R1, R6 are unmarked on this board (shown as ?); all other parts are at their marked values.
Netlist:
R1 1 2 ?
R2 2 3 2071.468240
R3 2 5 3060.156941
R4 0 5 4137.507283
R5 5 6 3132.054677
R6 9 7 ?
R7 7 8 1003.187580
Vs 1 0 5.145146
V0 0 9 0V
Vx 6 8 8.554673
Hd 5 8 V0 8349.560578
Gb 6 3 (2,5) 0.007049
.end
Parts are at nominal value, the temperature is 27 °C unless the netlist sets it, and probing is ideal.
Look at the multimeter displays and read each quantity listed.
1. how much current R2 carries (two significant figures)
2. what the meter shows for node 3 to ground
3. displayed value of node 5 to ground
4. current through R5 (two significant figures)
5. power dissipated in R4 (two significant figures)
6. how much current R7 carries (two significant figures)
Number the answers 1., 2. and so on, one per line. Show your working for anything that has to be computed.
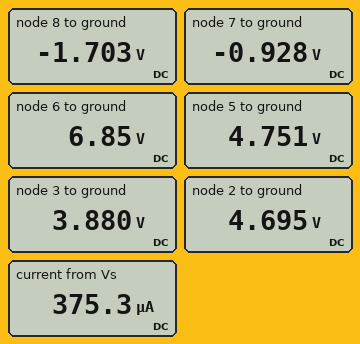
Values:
1. (4.695 V - 3.88 V) / 2.071 kΩ = 390 µA
2. 3.880 V
3. 4.751 V
4. (6.85 V - 4.751 V) / 3.132 kΩ = 670 µA
5. (4.751 V)^2 / 4.138 kΩ = 5.5 mW
6. (-928 mV - (-1.703 V)) / 1.003 kΩ = 770 µA
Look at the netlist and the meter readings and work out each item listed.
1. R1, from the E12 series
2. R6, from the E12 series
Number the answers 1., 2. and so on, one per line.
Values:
1. 1.2 kΩ
2. 1.2 kΩ
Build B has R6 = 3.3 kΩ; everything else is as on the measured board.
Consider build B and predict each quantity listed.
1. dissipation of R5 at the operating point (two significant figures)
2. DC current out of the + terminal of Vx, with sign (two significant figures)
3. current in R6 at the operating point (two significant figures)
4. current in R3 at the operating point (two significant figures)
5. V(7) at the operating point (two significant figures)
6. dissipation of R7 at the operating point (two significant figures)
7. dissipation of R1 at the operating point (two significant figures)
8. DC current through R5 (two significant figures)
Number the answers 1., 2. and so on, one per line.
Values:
1. 1.4 mW
2. -650 µA
3. 1.3 mA
4. 1.4 µA
5. -4.2 V
6. 1.6 mW
7. 950 nW
8. 680 µA
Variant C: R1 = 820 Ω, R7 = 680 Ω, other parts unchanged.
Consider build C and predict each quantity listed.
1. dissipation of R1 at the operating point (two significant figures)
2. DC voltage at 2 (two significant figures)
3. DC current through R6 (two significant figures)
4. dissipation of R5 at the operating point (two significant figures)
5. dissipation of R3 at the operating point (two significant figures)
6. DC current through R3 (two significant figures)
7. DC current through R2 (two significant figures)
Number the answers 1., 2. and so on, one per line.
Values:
1. 150 µW
2. 4.8 V
3. 750 µA
4. 1.7 mW
5. 1.3 µW
6. 21 µA
7. 440 µA
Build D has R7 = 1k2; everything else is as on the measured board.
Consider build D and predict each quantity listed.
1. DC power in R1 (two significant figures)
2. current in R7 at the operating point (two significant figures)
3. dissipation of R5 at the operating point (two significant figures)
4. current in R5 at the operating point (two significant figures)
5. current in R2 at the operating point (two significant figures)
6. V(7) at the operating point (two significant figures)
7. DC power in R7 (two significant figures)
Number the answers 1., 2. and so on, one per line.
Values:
1. 150 µW
2. 800 µA
3. 1.1 mW
4. 590 µA
5. 370 µA
6. -960 mV
7. 770 µW
